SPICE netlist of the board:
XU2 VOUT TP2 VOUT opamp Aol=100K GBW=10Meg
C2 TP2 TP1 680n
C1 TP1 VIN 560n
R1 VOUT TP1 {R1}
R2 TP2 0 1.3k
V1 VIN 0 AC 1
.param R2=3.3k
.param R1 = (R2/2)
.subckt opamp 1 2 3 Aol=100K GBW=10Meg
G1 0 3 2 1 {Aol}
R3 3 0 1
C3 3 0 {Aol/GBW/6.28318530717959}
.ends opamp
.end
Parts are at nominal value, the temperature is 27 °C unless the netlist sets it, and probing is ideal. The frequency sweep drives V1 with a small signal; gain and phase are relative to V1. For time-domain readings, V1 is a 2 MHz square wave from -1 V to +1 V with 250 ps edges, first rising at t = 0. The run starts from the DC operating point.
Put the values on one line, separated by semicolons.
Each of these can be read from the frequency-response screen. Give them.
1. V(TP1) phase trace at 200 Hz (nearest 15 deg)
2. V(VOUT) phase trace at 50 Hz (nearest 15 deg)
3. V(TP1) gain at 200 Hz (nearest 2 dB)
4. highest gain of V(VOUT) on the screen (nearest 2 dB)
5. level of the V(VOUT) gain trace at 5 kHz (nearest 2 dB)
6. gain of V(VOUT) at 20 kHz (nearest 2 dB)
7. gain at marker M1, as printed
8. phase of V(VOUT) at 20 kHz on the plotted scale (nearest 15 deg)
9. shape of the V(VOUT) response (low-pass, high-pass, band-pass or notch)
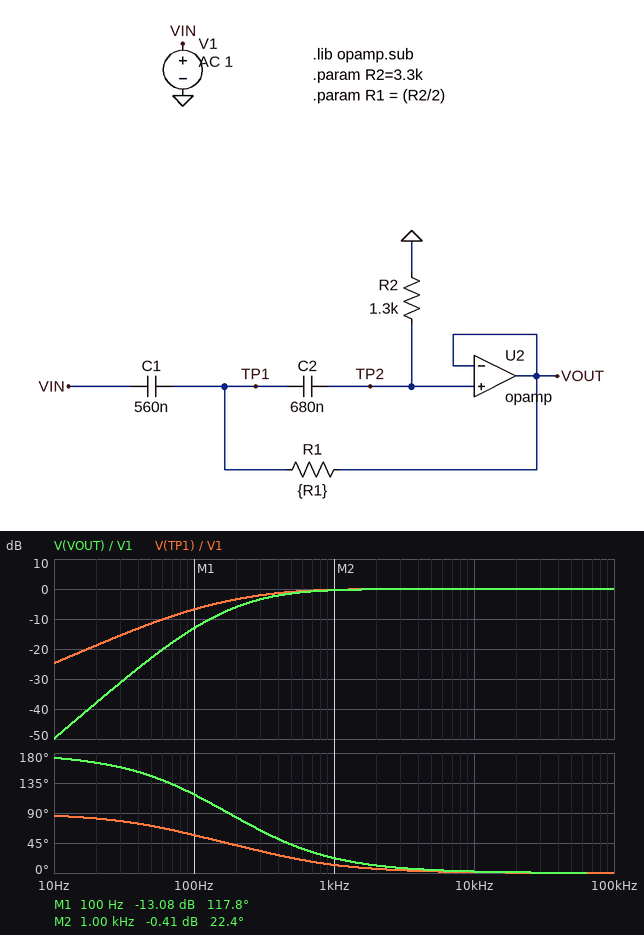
45 deg; 150 deg; -4 dB; 0 dB; 0 dB; 0 dB; -13.08 dB; 0 deg; high-pass
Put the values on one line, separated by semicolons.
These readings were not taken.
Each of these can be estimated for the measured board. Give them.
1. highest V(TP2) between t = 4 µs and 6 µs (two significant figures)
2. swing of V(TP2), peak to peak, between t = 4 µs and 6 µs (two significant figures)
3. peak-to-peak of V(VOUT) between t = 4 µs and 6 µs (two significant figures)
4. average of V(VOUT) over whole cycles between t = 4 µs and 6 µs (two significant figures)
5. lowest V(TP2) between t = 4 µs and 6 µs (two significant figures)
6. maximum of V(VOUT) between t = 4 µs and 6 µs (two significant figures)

2.0 V; 2.0 V; 2.0 V; 990 mV; -15 mV; 2.0 V
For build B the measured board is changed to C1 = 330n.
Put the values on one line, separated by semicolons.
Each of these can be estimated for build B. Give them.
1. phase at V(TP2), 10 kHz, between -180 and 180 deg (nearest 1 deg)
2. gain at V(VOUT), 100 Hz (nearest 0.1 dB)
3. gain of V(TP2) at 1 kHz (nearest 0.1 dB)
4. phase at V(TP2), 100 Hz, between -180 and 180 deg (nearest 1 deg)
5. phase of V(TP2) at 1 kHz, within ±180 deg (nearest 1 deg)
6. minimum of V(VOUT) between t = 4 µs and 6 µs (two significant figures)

3 deg; -16.9 dB; -0.8 dB; 128 deg; 30 deg; -21 mV
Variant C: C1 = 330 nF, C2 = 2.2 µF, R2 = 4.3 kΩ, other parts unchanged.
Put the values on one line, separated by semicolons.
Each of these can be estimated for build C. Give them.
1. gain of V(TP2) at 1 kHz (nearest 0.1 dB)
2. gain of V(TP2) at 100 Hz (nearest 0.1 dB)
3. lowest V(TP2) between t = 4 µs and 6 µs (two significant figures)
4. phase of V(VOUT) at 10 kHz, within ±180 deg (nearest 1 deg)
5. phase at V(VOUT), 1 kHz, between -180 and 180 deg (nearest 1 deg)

0 dB; -2.8 dB; -4.9 mV; 1 deg; 7 deg
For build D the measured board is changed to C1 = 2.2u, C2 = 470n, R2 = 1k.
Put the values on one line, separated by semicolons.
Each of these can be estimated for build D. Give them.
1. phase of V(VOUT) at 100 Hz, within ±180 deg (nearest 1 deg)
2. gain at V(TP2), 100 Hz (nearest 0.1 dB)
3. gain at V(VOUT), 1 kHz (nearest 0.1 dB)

97 deg; -12.3 dB; -0.6 dB
